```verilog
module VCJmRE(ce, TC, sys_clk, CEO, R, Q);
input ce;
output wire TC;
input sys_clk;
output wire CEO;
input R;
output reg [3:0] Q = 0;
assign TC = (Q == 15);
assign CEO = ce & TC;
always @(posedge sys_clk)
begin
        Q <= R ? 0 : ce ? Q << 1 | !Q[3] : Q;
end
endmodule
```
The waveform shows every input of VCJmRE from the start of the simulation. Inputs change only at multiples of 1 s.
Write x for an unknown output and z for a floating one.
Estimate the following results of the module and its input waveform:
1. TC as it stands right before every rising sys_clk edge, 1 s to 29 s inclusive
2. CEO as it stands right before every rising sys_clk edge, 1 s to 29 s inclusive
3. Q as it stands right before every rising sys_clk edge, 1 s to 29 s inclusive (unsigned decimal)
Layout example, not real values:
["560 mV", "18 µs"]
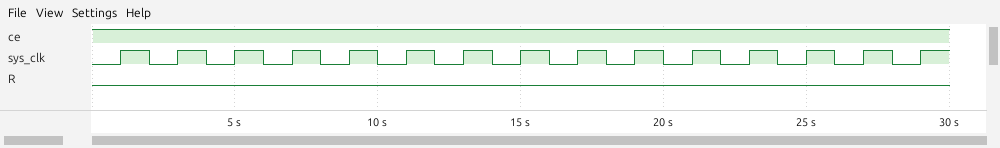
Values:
["0 0 0 0 1 0 0 0 0 0 0 0 1 0 0", "0 0 0 0 1 0 0 0 0 0 0 0 1 0 0", "0, 1, 3, 7, 15, 14, 12, 8, 0, 1, 3, 7, 15, 14, 12"]
